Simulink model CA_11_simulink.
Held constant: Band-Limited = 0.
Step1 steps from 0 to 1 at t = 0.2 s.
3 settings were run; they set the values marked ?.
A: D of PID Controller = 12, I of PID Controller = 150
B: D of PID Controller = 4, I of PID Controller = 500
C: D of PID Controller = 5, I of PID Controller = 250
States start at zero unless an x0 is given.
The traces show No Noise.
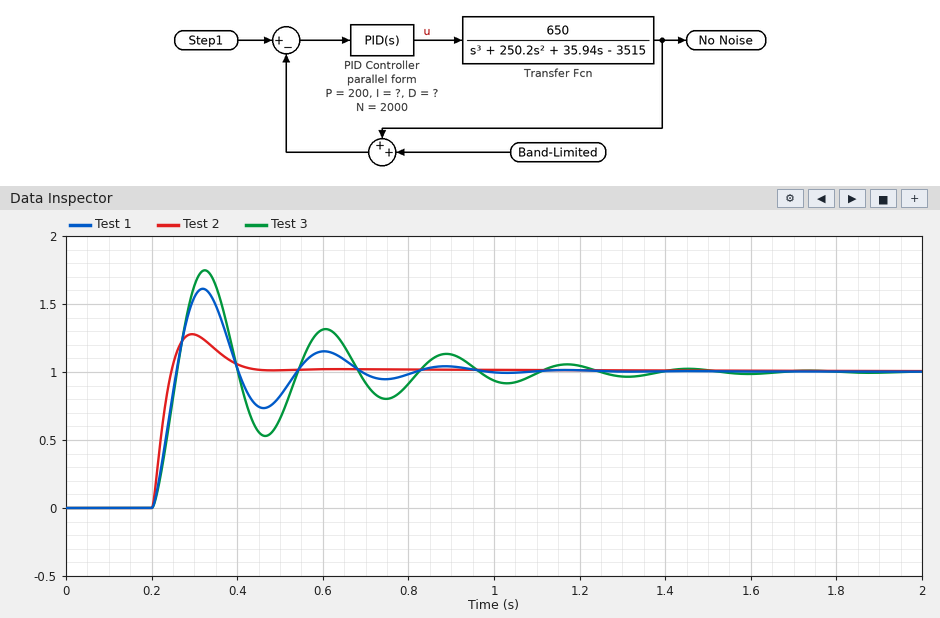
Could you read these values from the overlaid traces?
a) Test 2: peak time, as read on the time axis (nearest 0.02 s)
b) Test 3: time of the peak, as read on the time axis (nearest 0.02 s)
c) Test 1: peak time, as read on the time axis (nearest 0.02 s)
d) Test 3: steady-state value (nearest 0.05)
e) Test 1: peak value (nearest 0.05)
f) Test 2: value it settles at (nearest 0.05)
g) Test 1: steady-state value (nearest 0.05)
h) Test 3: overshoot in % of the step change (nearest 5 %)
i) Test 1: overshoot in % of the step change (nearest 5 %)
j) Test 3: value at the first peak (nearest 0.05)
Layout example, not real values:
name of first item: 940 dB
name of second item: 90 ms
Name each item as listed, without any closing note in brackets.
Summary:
Test 2: peak time, as read on the time axis: 0.30 s
Test 3: time of the peak, as read on the time axis: 0.32 s
Test 1: peak time, as read on the time axis: 0.32 s
Test 3: steady-state value: 1.00
Test 1: peak value: 1.60
Test 2: value it settles at: 1.00
Test 1: steady-state value: 1.00
Test 3: overshoot in % of the step change: 75 %
Test 1: overshoot in % of the step change: 60 %
Test 3: value at the first peak: 1.75
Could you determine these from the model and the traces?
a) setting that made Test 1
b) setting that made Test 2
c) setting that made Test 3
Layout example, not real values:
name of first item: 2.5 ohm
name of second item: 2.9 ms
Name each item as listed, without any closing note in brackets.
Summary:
setting that made Test 1: C
setting that made Test 2: A
setting that made Test 3: B
